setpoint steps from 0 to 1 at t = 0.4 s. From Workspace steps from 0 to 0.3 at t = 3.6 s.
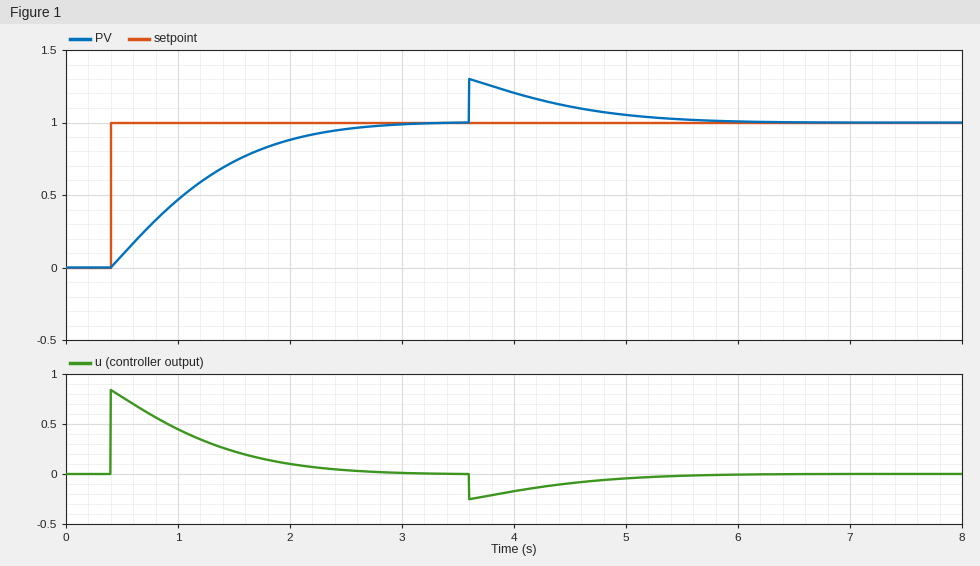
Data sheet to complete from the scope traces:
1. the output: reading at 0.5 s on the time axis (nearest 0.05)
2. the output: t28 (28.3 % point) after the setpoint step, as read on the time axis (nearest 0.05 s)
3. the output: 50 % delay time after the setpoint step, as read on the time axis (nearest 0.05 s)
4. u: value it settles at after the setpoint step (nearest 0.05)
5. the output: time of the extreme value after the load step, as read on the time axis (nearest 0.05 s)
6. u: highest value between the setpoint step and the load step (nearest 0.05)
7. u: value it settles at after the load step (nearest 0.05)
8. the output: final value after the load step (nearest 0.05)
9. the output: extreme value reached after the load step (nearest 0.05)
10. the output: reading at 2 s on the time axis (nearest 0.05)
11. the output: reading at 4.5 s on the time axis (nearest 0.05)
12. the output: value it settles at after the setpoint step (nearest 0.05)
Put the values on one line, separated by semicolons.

0.10; 0.75 s; 1.05 s; 0.00; 3.60 s; 0.85; 0.00; 1.00; 1.30; 0.90; 1.10; 1.00
